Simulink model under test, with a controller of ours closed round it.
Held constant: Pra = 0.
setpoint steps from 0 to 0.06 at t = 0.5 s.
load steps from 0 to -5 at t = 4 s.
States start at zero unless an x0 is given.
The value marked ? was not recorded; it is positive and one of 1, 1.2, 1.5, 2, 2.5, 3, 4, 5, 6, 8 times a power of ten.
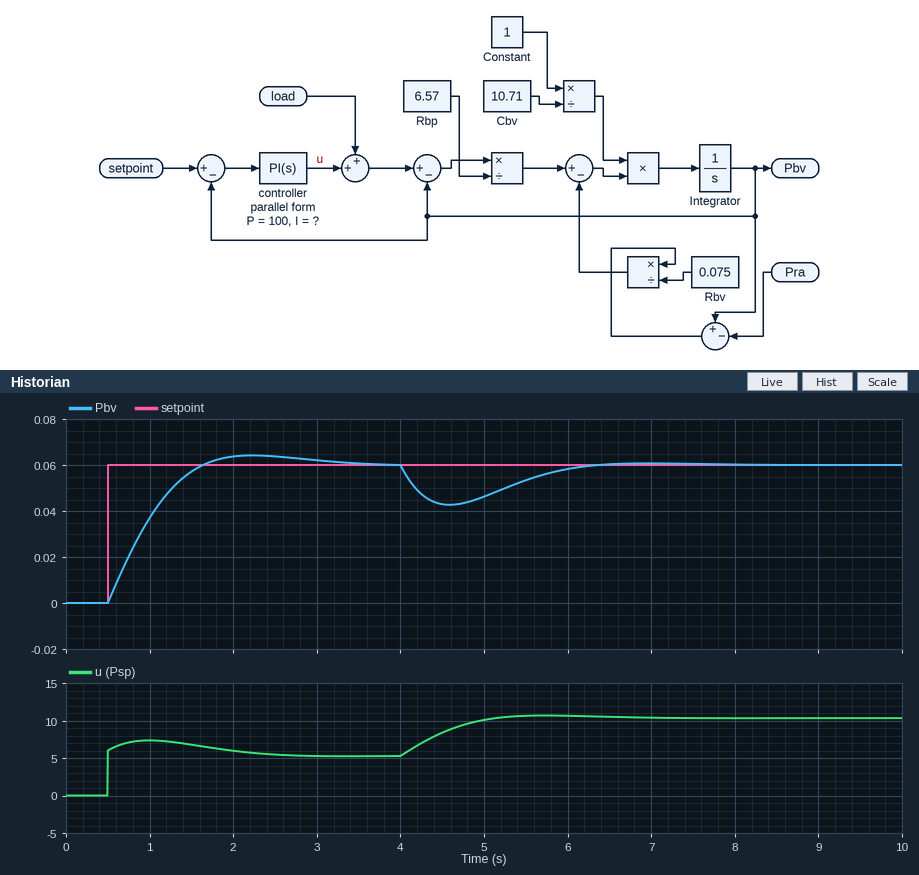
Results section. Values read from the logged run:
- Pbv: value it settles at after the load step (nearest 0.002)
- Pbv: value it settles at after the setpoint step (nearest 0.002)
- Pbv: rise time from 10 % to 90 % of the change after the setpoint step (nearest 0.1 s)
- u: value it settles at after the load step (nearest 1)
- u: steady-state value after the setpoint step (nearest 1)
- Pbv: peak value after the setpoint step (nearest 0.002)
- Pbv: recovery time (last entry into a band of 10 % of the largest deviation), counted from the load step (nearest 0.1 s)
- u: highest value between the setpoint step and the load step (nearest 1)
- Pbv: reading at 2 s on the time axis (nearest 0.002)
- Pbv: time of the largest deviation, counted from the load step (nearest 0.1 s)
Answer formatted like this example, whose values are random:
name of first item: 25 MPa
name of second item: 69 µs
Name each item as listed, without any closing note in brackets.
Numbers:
Pbv: value it settles at after the load step: 0.060
Pbv: value it settles at after the setpoint step: 0.060
Pbv: rise time from 10 % to 90 % of the change after the setpoint step: 0.8 s
u: value it settles at after the load step: 10
u: steady-state value after the setpoint step: 5
Pbv: peak value after the setpoint step: 0.064
Pbv: recovery time (last entry into a band of 10 % of the largest deviation), counted from the load step: 2.0 s
u: highest value between the setpoint step and the load step: 7
Pbv: reading at 2 s on the time axis: 0.064
Pbv: time of the largest deviation, counted from the load step: 0.6 s
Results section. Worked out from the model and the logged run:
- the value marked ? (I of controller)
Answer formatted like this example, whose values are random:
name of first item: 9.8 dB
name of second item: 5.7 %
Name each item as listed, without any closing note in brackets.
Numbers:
the value marked ?: 250
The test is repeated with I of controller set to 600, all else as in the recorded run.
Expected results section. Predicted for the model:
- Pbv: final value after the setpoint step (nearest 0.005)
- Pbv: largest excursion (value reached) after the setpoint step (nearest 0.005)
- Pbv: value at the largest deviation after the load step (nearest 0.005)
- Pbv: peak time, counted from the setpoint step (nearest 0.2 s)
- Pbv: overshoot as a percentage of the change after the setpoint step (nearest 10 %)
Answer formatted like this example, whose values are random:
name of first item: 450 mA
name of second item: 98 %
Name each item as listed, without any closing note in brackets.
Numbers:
Pbv: final value after the setpoint step: 0.060
Pbv: largest excursion (value reached) after the setpoint step: 0.075
Pbv: value at the largest deviation after the load step: 0.045
Pbv: peak time, counted from the setpoint step: 1.0 s
Pbv: overshoot as a percentage of the change after the setpoint step: 20 %
